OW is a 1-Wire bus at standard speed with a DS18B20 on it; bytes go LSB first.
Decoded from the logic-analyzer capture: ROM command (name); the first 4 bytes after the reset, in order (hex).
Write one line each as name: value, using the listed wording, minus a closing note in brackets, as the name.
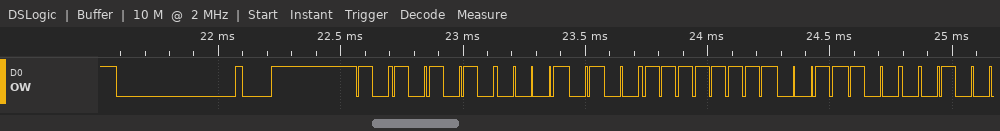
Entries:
ROM command: Match ROM
the first 4 bytes after the reset, in order: 55 28 FF 1C
